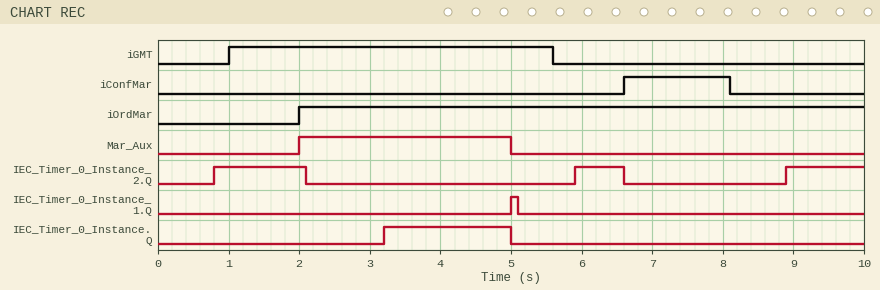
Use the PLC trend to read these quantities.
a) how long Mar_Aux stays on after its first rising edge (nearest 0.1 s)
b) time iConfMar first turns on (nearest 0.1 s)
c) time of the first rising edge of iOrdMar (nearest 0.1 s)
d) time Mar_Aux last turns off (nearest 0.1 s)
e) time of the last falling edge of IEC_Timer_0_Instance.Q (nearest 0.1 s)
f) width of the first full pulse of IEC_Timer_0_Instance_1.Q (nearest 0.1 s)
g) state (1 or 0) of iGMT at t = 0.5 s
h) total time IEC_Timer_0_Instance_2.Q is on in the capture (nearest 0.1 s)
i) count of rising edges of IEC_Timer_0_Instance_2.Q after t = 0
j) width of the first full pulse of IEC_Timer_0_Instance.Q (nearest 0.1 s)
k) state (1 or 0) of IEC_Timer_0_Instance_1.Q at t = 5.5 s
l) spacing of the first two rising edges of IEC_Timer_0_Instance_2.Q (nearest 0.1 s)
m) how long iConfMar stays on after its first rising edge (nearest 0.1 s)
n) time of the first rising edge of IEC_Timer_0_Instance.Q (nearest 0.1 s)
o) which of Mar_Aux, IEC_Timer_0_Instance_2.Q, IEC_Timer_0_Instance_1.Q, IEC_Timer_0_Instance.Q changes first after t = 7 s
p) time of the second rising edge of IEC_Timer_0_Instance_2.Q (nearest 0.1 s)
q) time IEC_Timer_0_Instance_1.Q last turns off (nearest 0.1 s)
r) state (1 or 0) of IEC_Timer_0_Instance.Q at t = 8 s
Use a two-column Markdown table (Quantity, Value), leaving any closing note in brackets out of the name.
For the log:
| Quantity | Value |
|---|---|
| how long Mar_Aux stays on after its first rising edge | 3.0 s |
| time iConfMar first turns on | 6.6 s |
| time of the first rising edge of iOrdMar | 2.0 s |
| time Mar_Aux last turns off | 5.0 s |
| time of the last falling edge of IEC_Timer_0_Instance.Q | 5.0 s |
| width of the first full pulse of IEC_Timer_0_Instance_1.Q | 0.1 s |
| state (1 or 0) of iGMT at t = 0.5 s | 0 |
| total time IEC_Timer_0_Instance_2.Q is on in the capture | 3.1 s |
| count of rising edges of IEC_Timer_0_Instance_2.Q after t = 0 | 3 |
| width of the first full pulse of IEC_Timer_0_Instance.Q | 1.8 s |
| state (1 or 0) of IEC_Timer_0_Instance_1.Q at t = 5.5 s | 0 |
| spacing of the first two rising edges of IEC_Timer_0_Instance_2.Q | 5.1 s |
| how long iConfMar stays on after its first rising edge | 1.5 s |
| time of the first rising edge of IEC_Timer_0_Instance.Q | 3.2 s |
| which of Mar_Aux, IEC_Timer_0_Instance_2.Q, IEC_Timer_0_Instance_1.Q, IEC_Timer_0_Instance.Q changes first after t = 7 s | IEC_Timer_0_Instance_2.Q |
| time of the second rising edge of IEC_Timer_0_Instance_2.Q | 5.9 s |
| time IEC_Timer_0_Instance_1.Q last turns off | 5.1 s |
| state (1 or 0) of IEC_Timer_0_Instance.Q at t = 8 s | 0 |
